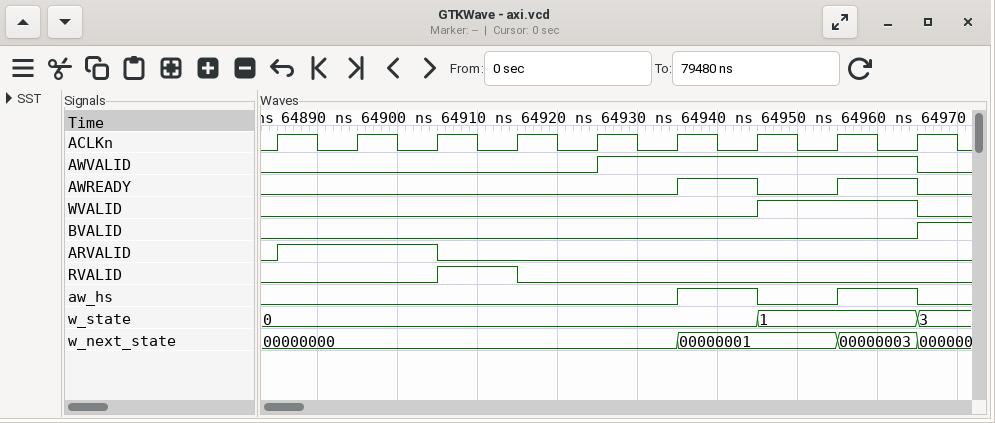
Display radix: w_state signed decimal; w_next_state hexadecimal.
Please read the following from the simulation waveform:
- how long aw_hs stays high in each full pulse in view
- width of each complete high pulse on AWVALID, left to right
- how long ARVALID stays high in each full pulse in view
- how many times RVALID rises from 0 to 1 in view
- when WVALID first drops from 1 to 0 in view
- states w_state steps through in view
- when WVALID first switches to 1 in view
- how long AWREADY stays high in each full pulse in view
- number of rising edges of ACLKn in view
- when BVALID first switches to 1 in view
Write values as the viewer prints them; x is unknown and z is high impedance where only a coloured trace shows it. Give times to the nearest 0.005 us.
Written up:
0.01 us, 0.01 us
0.04 us
0.02 us
1
64.965 us
0, 1, 3
64.945 us
0.01 us, 0.01 us
9
64.965 us
